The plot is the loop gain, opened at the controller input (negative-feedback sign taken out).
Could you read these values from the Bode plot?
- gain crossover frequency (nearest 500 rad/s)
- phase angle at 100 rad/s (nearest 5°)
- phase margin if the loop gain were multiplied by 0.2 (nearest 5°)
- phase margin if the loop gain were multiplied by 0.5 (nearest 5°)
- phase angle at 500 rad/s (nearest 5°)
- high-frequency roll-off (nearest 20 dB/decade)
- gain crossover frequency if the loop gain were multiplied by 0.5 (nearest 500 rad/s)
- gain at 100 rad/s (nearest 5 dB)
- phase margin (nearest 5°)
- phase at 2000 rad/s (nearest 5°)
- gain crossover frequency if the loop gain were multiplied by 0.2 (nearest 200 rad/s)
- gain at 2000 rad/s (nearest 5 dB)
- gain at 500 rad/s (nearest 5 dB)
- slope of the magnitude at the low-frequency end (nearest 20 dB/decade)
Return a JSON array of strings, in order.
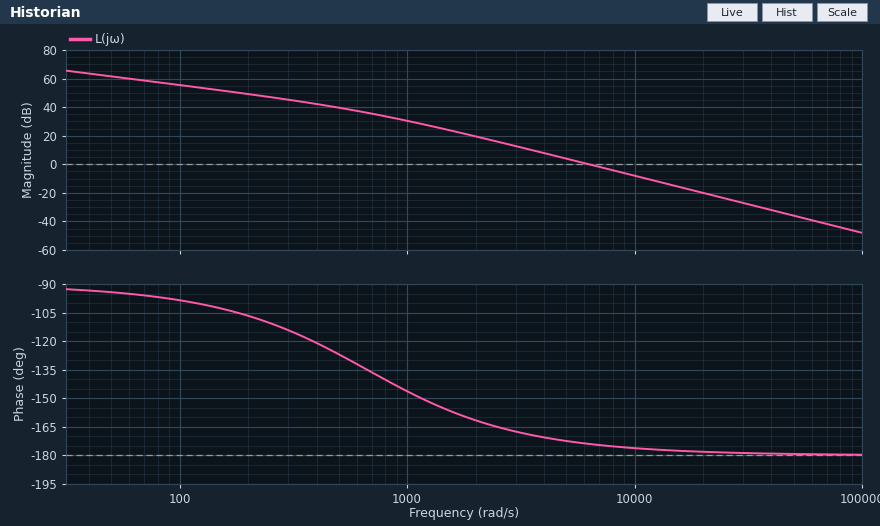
["6500 rad/s", "-100°", "15°", "10°", "-125°", "-40 dB/decade", "4500 rad/s", "55 dB", "5°", "-160°", "2800 rad/s", "20 dB", "40 dB", "-20 dB/decade"]
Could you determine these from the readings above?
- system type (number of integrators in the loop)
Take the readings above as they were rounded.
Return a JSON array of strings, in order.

["1"]
